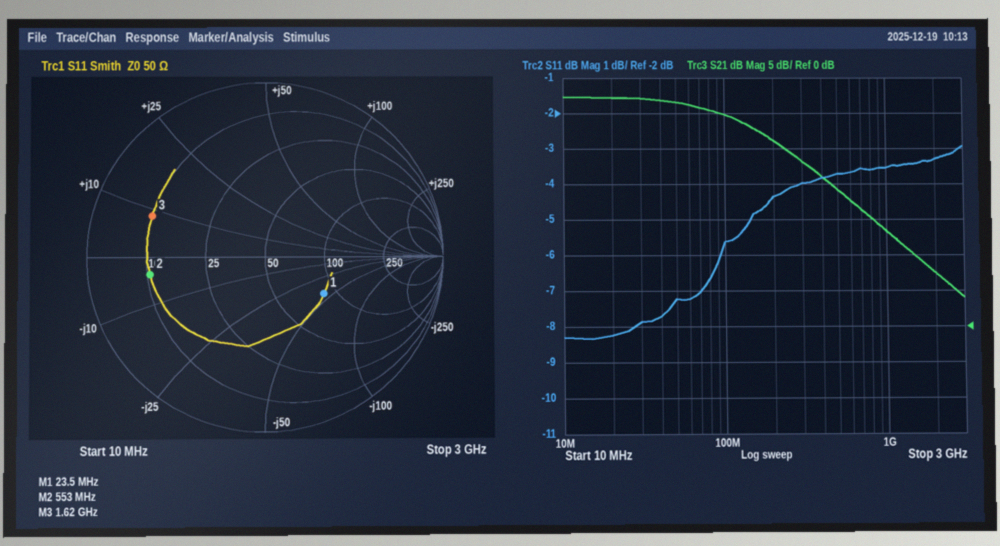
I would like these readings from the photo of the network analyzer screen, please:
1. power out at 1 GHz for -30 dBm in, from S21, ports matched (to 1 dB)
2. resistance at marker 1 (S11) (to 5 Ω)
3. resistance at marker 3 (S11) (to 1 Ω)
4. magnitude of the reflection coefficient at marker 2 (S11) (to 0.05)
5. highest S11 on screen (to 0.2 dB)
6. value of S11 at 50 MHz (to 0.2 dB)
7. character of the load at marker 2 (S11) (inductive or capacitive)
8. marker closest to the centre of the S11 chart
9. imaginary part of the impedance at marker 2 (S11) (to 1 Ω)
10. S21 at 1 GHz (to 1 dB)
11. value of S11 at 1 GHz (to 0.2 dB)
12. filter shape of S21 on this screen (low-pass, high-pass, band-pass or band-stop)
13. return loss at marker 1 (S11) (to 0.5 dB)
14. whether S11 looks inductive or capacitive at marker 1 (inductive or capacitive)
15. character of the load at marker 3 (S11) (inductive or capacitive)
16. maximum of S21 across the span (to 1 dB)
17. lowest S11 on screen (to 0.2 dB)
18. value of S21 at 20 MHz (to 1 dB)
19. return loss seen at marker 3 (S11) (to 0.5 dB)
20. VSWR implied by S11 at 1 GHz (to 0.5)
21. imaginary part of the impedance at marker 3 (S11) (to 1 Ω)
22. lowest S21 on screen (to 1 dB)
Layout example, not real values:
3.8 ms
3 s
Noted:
-17 dBm
85 Ω
10 Ω
0.65
-3.0 dB
-7.2 dB
capacitive
marker 1
-4 Ω
13 dB
-3.6 dB
low-pass
8.0 dB
capacitive
inductive
32 dB
-8.4 dB
32 dB
3.5 dB
5.0
+9 Ω
4 dB
